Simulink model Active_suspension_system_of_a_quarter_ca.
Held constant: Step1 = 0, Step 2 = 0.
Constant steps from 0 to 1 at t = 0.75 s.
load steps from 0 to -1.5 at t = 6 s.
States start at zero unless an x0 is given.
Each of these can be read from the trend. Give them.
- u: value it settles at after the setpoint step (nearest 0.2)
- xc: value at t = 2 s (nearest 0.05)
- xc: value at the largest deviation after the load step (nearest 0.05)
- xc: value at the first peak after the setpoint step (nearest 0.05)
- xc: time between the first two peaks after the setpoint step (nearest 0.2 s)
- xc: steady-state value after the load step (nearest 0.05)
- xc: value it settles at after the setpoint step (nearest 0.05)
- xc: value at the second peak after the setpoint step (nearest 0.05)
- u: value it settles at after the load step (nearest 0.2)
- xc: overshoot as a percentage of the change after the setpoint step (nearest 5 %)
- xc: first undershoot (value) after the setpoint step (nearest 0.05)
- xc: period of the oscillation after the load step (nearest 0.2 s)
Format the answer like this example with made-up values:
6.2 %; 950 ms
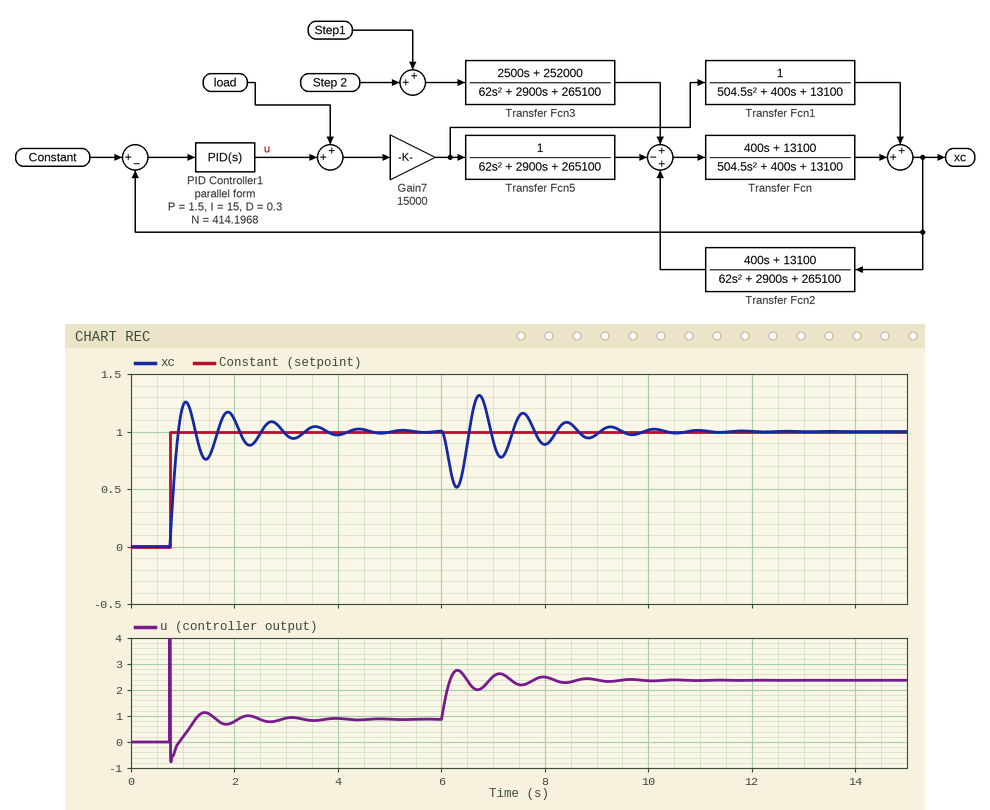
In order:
0.8; 1.10; 0.50; 1.25; 0.8 s; 1.00; 1.00; 1.15; 2.4; 25 %; 0.75; 0.8 s
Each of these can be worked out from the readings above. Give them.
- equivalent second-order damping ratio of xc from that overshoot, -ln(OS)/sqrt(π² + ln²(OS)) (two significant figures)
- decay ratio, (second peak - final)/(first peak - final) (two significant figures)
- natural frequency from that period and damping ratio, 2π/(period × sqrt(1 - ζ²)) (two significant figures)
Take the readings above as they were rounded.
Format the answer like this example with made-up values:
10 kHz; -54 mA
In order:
0.40; 0.60; 8.6 rad/s
